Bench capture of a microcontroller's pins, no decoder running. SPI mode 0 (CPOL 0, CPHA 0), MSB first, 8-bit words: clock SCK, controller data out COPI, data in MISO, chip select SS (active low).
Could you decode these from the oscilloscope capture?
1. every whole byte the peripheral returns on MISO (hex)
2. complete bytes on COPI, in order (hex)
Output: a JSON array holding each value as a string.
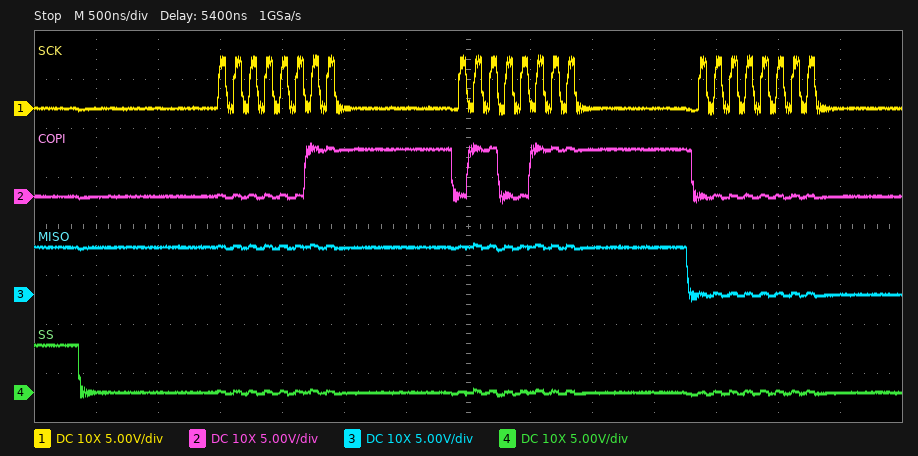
["0xFF 0xFF 0x00", "0x03 0x67 0x00"]
